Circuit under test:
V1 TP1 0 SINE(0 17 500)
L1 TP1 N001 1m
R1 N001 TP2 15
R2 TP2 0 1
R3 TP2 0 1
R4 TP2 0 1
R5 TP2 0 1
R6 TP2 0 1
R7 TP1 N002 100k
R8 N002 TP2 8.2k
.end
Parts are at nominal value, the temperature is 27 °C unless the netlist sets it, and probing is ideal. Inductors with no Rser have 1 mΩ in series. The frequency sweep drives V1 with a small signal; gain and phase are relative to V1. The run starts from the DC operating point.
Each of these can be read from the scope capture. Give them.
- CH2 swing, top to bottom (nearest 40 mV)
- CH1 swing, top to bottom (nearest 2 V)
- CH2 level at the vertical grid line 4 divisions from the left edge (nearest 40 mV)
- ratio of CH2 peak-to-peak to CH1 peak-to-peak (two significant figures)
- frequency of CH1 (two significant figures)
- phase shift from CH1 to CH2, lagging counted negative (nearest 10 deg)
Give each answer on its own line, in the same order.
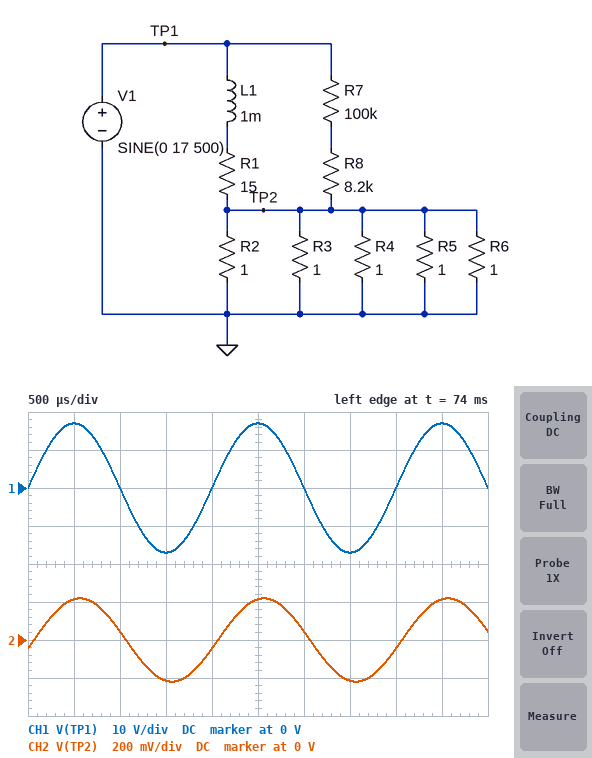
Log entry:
440 mV
34 V
-40 mV
0.013
500 Hz
-10 deg
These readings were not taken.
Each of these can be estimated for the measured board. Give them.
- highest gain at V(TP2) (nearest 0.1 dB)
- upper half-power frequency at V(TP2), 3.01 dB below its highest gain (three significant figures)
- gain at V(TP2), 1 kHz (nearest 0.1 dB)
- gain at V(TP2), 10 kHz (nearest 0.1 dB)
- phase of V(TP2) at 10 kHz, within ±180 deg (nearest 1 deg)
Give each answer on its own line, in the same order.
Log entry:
-37.6 dB
2.42 kHz
-38.3 dB
-50.2 dB
-76 deg
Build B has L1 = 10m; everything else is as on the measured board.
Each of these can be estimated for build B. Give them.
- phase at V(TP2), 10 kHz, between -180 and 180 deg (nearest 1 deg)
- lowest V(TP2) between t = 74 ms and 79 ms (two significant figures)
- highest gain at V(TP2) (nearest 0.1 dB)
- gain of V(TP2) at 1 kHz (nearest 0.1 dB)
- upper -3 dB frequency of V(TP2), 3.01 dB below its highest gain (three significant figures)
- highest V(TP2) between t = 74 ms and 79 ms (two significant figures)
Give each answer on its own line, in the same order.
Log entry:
-88 deg
-97 mV
-37.6 dB
-50.2 dB
242 Hz
97 mV
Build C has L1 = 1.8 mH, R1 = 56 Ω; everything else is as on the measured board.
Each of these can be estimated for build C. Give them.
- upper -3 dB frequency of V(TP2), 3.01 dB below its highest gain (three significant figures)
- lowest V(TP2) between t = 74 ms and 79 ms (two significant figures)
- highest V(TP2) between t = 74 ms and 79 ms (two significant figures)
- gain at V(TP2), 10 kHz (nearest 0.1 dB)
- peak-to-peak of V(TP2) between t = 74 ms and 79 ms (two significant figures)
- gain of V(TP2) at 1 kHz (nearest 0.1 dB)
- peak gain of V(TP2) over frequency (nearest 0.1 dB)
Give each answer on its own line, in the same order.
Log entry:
4.97 kHz
-60 mV
60 mV
-56.0 dB
120 mV
-49.1 dB
-49.0 dB
